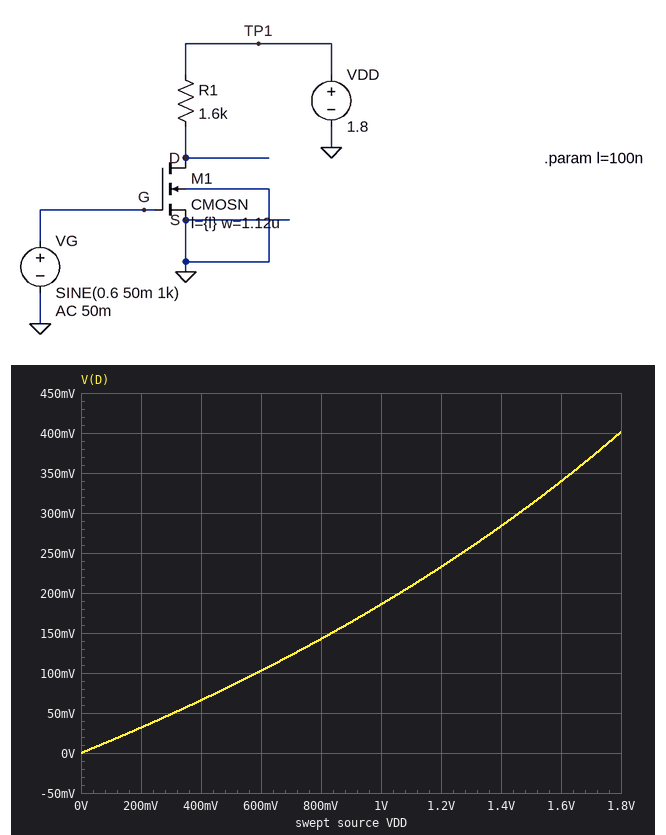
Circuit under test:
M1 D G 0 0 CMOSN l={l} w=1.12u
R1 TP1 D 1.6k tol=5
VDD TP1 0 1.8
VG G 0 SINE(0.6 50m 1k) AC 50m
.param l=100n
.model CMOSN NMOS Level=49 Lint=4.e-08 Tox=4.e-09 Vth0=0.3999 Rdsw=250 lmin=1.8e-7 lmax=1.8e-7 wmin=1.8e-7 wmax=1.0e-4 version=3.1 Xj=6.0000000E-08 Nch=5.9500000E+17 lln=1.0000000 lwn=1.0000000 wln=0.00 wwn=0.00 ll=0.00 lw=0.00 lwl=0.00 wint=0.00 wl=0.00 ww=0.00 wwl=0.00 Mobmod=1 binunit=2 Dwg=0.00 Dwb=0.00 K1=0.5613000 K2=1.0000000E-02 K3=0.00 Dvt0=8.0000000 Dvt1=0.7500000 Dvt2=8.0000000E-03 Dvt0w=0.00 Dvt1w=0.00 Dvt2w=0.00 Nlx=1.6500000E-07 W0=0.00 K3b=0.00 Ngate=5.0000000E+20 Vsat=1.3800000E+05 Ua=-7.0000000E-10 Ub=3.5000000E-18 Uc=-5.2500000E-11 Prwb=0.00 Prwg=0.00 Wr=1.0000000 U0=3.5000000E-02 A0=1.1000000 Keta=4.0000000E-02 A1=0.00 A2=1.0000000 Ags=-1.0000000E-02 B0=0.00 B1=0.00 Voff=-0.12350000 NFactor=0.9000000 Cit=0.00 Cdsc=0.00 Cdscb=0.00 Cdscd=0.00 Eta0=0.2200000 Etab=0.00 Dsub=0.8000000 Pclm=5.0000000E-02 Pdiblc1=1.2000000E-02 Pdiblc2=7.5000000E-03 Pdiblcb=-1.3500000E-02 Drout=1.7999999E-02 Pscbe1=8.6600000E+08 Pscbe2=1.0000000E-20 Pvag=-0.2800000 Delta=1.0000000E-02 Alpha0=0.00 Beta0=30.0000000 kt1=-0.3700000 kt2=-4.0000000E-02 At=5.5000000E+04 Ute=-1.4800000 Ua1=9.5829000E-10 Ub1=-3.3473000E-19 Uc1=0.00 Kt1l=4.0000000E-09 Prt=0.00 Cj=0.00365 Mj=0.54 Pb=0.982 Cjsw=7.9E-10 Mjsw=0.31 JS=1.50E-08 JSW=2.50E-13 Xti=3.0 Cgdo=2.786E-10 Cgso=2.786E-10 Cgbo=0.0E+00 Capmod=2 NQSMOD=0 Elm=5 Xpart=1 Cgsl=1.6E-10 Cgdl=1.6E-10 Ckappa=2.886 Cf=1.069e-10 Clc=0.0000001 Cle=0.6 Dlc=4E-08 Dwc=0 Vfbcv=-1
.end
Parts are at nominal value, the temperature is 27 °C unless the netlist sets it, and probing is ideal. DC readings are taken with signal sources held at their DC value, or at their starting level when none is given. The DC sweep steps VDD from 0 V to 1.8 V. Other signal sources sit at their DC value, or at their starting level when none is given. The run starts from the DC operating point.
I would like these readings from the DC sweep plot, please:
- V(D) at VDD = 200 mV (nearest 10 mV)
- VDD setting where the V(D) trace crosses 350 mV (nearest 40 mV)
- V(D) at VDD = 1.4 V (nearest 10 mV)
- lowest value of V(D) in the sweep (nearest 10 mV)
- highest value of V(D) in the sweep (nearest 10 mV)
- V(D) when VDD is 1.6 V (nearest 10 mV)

30 mV
1.64 V
280 mV
0 V
400 mV
340 mV
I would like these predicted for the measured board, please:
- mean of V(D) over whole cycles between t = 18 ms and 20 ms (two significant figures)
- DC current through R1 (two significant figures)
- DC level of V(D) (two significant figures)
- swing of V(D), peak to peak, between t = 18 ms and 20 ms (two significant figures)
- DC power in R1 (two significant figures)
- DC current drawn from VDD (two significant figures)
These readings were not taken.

400 mV
870 µA
400 mV
26 mV
1.2 mW
870 µA
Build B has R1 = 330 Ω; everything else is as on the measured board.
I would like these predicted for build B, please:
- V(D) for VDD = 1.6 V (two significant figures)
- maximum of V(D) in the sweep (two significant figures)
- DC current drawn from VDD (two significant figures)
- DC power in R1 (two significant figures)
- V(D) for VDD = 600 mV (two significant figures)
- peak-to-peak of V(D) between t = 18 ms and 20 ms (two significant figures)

1.1 V
1.3 V
1.6 mA
870 µW
340 mV
20 mV
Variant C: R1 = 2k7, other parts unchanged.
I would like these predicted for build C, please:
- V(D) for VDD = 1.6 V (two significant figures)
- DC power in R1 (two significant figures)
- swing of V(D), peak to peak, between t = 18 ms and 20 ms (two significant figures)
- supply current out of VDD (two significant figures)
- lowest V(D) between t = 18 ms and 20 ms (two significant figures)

190 mV
920 µW
11 mV
580 µA
220 mV
